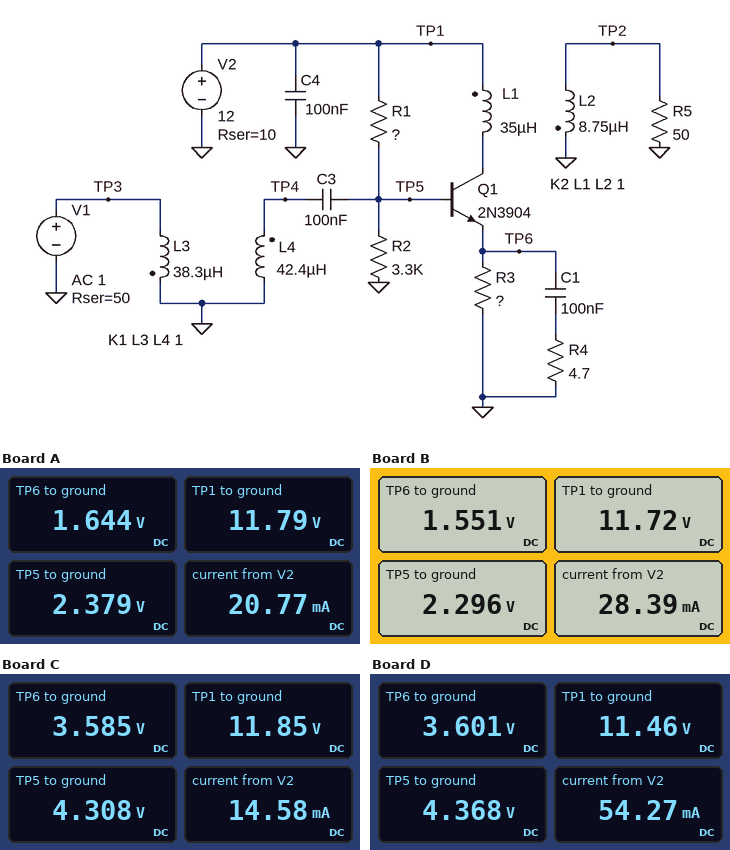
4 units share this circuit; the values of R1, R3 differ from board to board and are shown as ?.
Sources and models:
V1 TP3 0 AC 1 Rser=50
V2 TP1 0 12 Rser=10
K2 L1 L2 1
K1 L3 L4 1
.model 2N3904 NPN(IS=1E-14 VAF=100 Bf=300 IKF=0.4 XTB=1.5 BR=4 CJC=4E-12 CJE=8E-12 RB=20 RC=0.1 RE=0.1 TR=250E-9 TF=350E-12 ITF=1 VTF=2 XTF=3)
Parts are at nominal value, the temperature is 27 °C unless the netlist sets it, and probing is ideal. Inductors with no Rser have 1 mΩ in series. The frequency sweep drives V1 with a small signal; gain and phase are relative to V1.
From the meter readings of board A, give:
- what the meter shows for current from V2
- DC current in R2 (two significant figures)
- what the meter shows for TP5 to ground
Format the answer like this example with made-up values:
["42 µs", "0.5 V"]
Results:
["20.77 mA", "720 µA", "2.379 V"]
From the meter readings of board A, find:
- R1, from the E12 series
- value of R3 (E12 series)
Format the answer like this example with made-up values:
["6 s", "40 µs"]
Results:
["12 kΩ", "82 Ω"]
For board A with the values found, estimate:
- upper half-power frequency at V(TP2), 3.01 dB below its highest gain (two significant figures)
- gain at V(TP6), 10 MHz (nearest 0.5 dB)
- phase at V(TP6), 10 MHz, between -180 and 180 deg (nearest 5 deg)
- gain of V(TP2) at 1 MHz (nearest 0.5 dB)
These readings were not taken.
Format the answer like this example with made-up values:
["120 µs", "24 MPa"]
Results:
["19 MHz", "-3.5 dB", "150 deg", "21.5 dB"]
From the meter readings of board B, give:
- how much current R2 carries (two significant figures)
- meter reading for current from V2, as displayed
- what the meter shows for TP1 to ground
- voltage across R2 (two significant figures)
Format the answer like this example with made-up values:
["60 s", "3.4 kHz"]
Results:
["700 µA", "28.39 mA", "11.72 V", "2.3 V"]
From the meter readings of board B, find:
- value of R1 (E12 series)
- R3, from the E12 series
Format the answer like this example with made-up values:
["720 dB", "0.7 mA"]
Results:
["12 kΩ", "56 Ω"]
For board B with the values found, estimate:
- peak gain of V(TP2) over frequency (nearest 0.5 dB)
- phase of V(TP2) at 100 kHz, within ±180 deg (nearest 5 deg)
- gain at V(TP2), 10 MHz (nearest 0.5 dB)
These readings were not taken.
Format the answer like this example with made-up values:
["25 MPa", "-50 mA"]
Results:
["25.0 dB", "-155 deg", "24.0 dB"]
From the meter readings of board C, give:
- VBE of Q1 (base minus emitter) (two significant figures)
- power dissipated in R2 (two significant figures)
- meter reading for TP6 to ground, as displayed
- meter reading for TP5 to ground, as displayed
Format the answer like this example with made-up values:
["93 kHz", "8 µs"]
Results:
["720 mV", "5.6 mW", "3.585 V", "4.308 V"]
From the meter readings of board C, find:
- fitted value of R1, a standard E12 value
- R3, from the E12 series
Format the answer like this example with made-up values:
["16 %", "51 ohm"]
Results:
["5.6 kΩ", "270 Ω"]
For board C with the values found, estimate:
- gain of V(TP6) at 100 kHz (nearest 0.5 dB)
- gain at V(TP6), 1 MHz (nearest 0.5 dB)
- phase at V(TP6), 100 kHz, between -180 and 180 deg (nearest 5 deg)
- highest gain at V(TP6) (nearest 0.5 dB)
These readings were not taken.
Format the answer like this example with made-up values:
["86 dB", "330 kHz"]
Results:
["-7.5 dB", "-3.0 dB", "-125 deg", "-3.0 dB"]
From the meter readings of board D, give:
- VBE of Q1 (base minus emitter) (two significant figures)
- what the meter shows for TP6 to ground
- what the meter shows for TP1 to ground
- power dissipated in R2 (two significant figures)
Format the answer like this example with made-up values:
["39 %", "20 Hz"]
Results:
["770 mV", "3.601 V", "11.46 V", "5.8 mW"]
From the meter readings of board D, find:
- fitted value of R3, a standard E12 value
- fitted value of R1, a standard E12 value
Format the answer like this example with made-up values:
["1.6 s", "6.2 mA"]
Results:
["68 Ω", "4.7 kΩ"]
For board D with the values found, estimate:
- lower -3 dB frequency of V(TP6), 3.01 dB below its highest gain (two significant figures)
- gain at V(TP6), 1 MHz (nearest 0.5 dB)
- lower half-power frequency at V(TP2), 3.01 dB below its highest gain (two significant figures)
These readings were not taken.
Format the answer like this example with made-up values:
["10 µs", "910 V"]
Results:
["160 kHz", "-1.5 dB", "940 kHz"]
